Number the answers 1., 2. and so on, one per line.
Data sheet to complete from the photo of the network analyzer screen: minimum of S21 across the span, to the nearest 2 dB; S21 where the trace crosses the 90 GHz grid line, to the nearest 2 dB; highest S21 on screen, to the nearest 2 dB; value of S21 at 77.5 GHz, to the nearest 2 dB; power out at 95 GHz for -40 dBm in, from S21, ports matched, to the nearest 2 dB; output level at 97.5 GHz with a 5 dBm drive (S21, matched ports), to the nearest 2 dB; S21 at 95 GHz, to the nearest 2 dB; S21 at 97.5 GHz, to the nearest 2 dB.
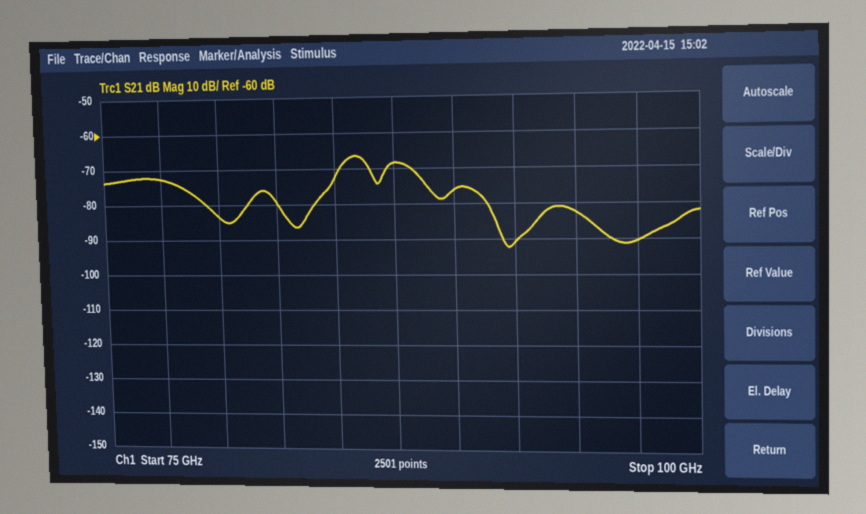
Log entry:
1. -92 dB
2. -76 dB
3. -66 dB
4. -72 dB
5. -122 dBm
6. -86 dBm
7. -82 dB
8. -90 dB
